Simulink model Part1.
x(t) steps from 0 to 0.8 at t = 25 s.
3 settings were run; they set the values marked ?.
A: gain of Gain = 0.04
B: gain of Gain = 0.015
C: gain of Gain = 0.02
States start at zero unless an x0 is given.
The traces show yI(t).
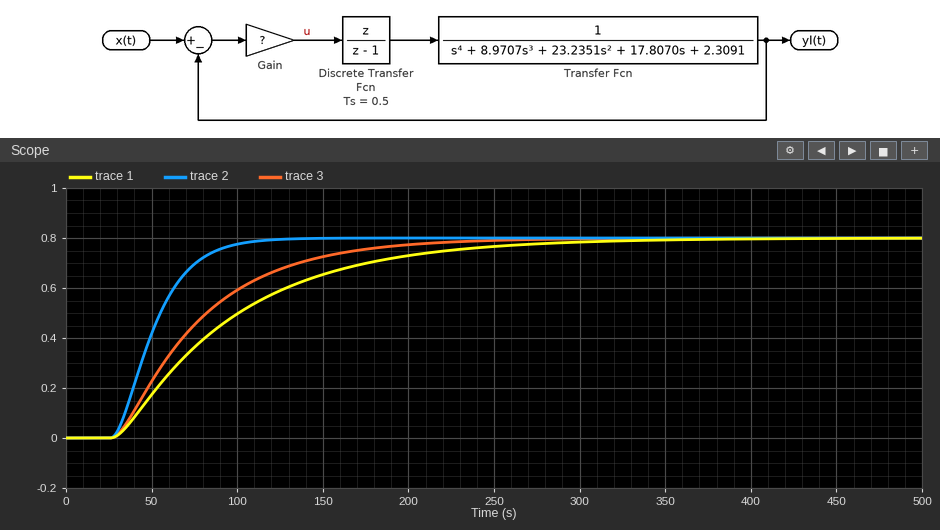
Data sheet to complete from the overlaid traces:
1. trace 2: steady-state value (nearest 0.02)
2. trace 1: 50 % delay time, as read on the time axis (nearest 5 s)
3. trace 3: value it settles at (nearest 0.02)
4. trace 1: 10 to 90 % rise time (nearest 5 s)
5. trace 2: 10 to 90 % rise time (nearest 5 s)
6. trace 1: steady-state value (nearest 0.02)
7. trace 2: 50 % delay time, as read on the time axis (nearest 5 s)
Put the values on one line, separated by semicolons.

0.80; 80 s; 0.80; 150 s; 45 s; 0.80; 50 s
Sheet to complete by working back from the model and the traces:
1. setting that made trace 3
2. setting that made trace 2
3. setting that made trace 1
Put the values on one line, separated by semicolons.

C; A; B
